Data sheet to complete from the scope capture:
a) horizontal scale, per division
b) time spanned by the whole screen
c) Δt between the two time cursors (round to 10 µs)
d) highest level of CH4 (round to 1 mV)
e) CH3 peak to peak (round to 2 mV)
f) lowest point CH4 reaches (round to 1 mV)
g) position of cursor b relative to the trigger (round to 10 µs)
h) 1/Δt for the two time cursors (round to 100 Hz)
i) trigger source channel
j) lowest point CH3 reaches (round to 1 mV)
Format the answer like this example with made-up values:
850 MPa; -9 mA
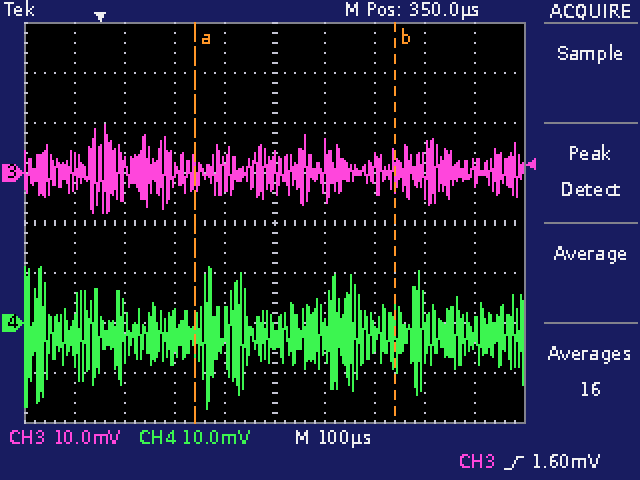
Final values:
100 µs; 1 ms; 400 µs; 11 mV; 18 mV; -17 mV; +590 µs; 2.5 kHz; CH3; -8 mV
